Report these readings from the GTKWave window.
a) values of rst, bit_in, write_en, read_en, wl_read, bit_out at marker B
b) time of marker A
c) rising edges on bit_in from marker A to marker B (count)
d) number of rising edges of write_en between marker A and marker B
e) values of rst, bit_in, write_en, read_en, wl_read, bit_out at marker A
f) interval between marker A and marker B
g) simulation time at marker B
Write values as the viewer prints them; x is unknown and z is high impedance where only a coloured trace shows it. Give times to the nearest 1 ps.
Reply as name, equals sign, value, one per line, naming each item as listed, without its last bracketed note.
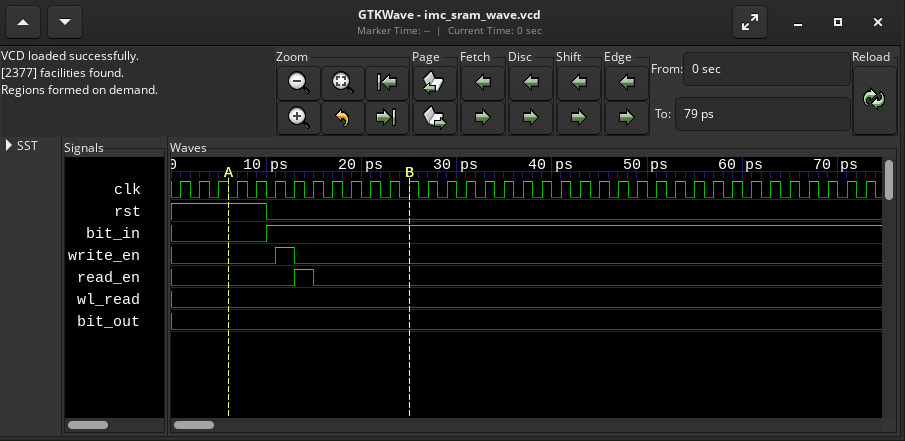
values of rst, bit_in, write_en, read_en, wl_read, bit_out at marker B = rst=0, bit_in=1, write_en=0, read_en=0, wl_read=0, bit_out=0
time of marker A = 6 ps
rising edges on bit_in from marker A to marker B = 1
number of rising edges of write_en between marker A and marker B = 1
values of rst, bit_in, write_en, read_en, wl_read, bit_out at marker A = rst=1, bit_in=0, write_en=0, read_en=0, wl_read=0, bit_out=0
interval between marker A and marker B = 19 ps
simulation time at marker B = 25 ps
